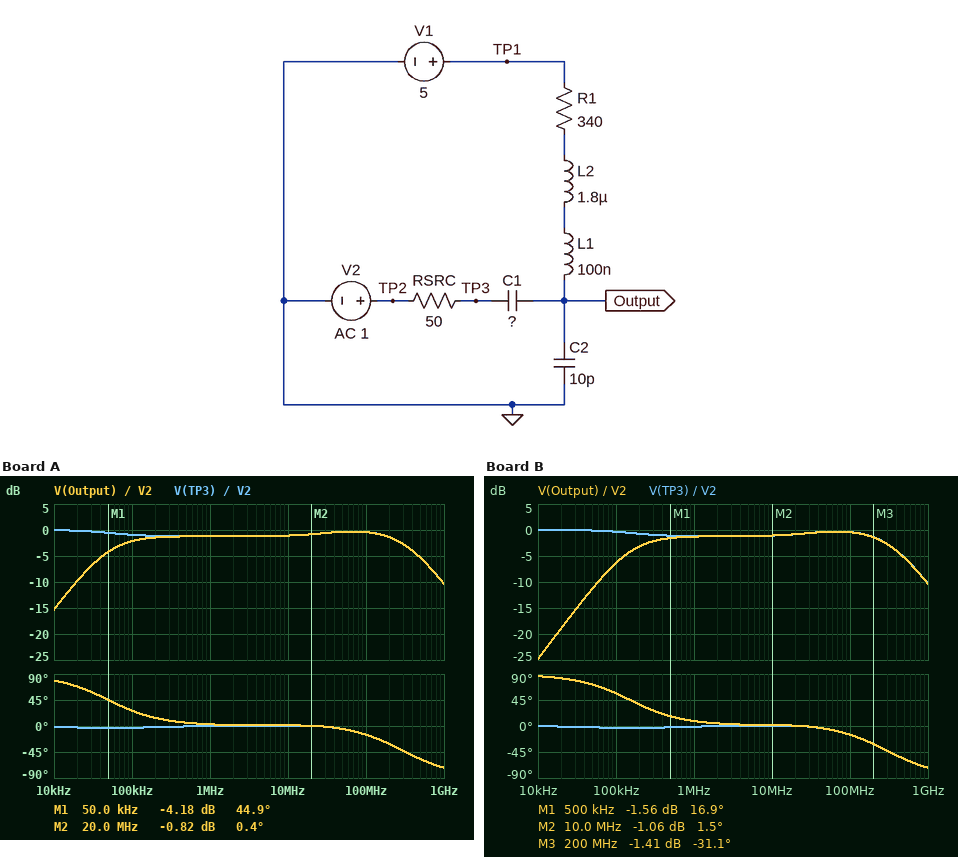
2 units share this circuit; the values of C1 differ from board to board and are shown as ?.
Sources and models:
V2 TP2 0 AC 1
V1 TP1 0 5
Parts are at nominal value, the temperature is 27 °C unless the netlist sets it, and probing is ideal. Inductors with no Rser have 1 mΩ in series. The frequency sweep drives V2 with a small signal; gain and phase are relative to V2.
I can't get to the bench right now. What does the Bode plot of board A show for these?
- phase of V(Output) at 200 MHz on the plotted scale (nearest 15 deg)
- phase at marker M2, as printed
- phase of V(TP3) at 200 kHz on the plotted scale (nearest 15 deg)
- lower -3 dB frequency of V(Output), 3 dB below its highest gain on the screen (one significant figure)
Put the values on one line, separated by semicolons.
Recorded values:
-30 deg; 0.4 deg; 0 deg; 60 kHz
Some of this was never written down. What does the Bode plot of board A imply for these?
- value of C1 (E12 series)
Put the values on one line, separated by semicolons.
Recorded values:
8.2 nF
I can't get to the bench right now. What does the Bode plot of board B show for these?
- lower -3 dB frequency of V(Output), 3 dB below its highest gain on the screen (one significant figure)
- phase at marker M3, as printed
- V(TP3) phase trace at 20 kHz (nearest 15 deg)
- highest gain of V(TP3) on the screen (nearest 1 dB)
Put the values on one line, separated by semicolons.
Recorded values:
200 kHz; -31.1 deg; 0 deg; 0 dB
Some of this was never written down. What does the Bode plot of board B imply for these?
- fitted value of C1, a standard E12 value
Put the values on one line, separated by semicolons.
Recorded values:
2.7 nF
